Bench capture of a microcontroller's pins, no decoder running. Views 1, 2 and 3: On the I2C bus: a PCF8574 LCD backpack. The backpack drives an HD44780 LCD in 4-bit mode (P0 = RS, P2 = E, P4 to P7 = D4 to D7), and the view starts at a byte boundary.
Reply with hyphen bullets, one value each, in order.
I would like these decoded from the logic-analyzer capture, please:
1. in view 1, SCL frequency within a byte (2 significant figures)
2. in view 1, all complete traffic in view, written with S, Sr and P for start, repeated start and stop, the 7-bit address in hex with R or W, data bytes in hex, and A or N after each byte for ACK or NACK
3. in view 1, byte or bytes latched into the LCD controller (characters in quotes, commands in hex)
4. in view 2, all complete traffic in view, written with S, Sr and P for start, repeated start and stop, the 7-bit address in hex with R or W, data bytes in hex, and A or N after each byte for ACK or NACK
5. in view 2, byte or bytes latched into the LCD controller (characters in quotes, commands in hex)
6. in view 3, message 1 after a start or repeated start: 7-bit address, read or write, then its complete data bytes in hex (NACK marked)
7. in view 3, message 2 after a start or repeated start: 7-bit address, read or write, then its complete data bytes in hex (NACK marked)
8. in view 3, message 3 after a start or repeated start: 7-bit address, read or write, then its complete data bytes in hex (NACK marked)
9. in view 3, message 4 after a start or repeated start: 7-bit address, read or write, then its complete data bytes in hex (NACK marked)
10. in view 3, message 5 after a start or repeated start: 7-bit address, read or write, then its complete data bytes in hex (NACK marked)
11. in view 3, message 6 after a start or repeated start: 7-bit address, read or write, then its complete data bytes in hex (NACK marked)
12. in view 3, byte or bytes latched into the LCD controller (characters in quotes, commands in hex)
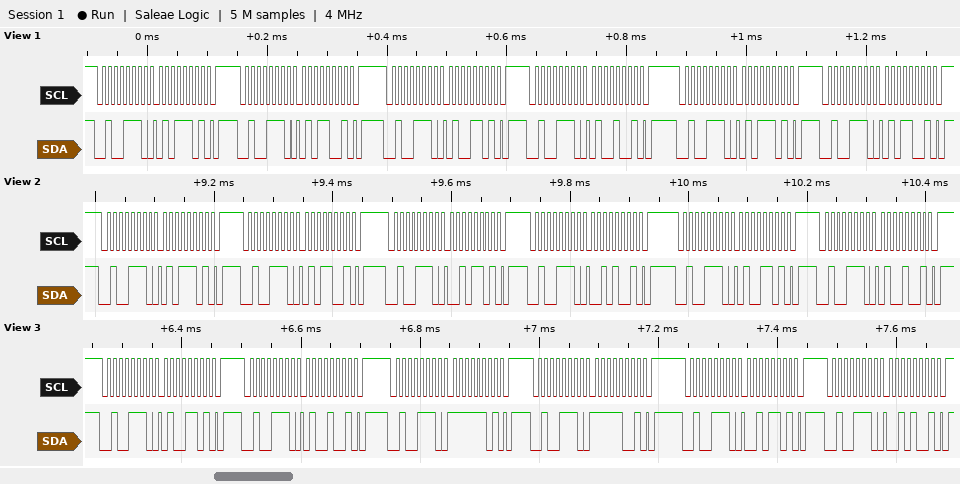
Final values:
- 100 kHz
- S 27W A 5D A P S 27W A 59 A P S 27W A 4D A P S 27W A 49 A P S 27W A 5D A P S 27W A 59 A P
- 'T'
- S 27W A 5D A P S 27W A 59 A P S 27W A 2D A P S 27W A 29 A P S 27W A 4D A P S 27W A 49 A P
- 'R'
- 0x27 write: 4D
- 0x27 write: 49
- 0x27 write: FD
- 0x27 write: F9
- 0x27 write: 2D
- 0x27 write: 29
- 'O'
